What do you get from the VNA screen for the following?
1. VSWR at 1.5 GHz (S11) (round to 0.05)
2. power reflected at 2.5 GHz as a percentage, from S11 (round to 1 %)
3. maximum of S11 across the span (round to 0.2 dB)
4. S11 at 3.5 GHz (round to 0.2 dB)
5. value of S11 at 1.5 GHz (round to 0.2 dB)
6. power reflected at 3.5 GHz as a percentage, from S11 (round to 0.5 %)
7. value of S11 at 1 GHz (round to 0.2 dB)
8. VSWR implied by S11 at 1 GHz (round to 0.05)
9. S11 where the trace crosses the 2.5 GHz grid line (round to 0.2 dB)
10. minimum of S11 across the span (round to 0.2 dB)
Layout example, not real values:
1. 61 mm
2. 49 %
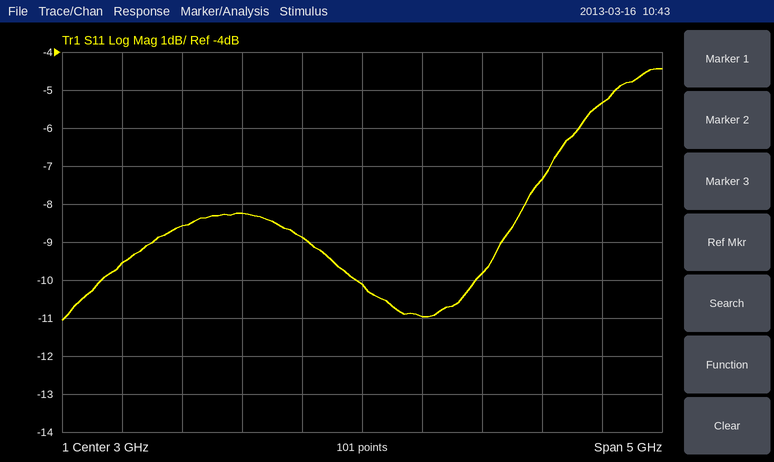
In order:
1. 2.20
2. 13 %
3. -4.4 dB
4. -11.0 dB
5. -8.6 dB
6. 8.0 %
7. -9.6 dB
8. 2.00
9. -8.8 dB
10. -11.0 dB
